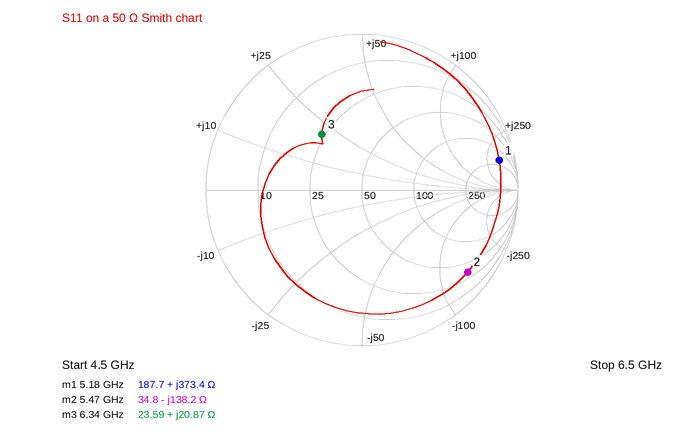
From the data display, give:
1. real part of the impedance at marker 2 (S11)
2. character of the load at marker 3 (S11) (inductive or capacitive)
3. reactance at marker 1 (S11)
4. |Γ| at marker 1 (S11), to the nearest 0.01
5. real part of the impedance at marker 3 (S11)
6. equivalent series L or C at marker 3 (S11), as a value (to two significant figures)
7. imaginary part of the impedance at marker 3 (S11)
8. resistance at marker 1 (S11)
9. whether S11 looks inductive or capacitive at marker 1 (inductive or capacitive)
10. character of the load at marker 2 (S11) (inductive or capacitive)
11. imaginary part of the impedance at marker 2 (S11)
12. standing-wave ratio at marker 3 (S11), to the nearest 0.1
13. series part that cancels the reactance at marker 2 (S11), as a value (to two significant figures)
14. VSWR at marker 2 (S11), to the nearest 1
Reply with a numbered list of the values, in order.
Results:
1. 34.8 Ω
2. inductive
3. +373.4 Ω
4. 0.90
5. 23.59 Ω
6. 520 pH
7. +20.87 Ω
8. 187.7 Ω
9. inductive
10. capacitive
11. -138.2 Ω
12. 2.6
13. 4.0 nH
14. 13
